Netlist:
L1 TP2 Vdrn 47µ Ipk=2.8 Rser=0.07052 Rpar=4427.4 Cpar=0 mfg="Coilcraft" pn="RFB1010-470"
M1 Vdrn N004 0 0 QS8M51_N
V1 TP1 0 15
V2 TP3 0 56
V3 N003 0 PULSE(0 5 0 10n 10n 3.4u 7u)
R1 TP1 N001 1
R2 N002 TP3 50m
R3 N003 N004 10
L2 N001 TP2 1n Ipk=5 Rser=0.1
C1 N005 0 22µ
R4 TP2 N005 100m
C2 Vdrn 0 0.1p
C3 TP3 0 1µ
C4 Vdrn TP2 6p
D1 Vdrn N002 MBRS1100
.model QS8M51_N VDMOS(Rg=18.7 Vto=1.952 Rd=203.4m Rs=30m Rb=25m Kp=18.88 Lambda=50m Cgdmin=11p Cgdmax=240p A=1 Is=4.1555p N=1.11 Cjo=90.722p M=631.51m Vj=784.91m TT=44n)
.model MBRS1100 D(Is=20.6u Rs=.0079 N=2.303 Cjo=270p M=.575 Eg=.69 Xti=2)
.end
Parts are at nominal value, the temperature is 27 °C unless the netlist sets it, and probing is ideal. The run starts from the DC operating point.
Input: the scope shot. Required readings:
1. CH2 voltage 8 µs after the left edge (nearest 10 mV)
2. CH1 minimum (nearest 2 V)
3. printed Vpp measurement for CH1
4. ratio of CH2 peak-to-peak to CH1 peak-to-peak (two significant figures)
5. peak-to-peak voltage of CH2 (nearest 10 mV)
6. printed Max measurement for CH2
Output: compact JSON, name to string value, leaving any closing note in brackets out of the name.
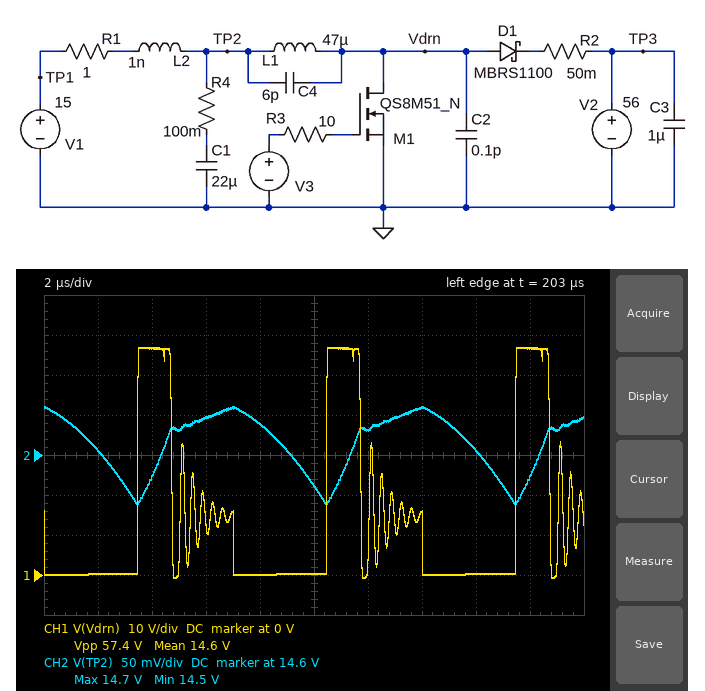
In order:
{"CH2 voltage 8 µs after the left edge": "14.64 V", "CH1 minimum": "0 V", "printed Vpp measurement for CH1": "57.4 V", "ratio of CH2 peak-to-peak to CH1 peak-to-peak": "0.0021", "peak-to-peak voltage of CH2": "120 mV", "printed Max measurement for CH2": "14.7 V"}
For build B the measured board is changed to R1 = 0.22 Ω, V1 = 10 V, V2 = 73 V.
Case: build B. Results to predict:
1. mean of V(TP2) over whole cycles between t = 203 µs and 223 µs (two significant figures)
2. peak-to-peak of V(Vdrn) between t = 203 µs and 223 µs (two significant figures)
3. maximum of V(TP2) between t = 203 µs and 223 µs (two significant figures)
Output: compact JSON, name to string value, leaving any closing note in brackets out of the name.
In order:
{"mean of V(TP2) over whole cycles between t = 203 µs and 223 µs": "9.9 V", "peak-to-peak of V(Vdrn) between t = 203 µs and 223 µs": "74 V", "maximum of V(TP2) between t = 203 µs and 223 µs": "10 V"}
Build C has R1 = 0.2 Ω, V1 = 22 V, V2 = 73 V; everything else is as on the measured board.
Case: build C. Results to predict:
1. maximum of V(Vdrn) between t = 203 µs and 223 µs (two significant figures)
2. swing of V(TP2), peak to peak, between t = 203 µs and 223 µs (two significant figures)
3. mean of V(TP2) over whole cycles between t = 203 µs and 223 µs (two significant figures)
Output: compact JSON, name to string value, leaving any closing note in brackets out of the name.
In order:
{"maximum of V(Vdrn) between t = 203 µs and 223 µs": "74 V", "swing of V(TP2), peak to peak, between t = 203 µs and 223 µs": "140 mV", "mean of V(TP2) over whole cycles between t = 203 µs and 223 µs": "22 V"}
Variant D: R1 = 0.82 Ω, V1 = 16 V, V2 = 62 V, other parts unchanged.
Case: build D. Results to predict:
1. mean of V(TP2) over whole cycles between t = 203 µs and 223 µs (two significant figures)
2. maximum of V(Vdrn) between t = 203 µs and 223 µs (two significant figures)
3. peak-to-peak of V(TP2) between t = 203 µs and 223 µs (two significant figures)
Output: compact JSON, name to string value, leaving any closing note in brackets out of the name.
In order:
{"mean of V(TP2) over whole cycles between t = 203 µs and 223 µs": "16 V", "maximum of V(Vdrn) between t = 203 µs and 223 µs": "63 V", "peak-to-peak of V(TP2) between t = 203 µs and 223 µs": "130 mV"}
